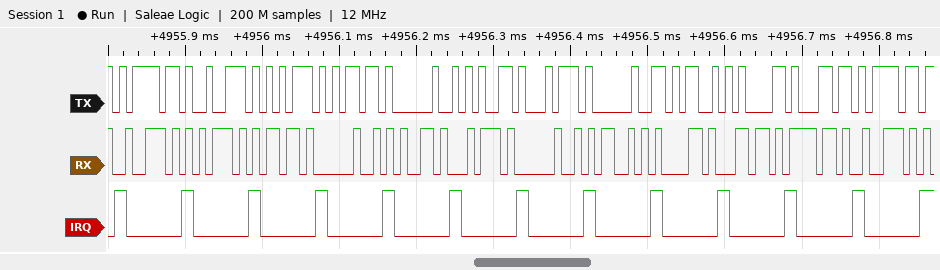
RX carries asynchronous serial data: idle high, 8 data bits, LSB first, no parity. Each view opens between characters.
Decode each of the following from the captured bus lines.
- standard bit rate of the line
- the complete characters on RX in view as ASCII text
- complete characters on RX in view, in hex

115200 baud
"rum et Malor"
72, 75, 6D, 20, 65, 74, 20, 4D, 61, 6C, 6F, 72
